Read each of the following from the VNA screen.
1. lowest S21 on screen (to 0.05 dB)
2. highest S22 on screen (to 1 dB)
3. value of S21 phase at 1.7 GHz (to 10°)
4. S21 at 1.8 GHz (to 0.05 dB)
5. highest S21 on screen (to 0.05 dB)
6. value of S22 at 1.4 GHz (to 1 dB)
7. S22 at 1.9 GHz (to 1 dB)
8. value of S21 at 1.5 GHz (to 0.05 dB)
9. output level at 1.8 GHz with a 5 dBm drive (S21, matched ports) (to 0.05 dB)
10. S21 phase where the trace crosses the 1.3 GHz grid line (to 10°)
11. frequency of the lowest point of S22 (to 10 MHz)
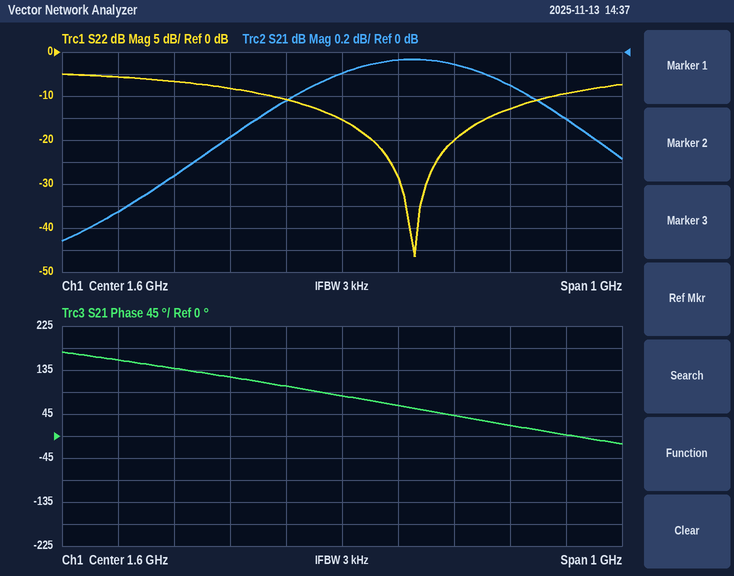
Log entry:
-1.70 dB
-5 dB
60°
-0.10 dB
-0.05 dB
-8 dB
-13 dB
-0.45 dB
4.90 dBm
140°
1.73 GHz
